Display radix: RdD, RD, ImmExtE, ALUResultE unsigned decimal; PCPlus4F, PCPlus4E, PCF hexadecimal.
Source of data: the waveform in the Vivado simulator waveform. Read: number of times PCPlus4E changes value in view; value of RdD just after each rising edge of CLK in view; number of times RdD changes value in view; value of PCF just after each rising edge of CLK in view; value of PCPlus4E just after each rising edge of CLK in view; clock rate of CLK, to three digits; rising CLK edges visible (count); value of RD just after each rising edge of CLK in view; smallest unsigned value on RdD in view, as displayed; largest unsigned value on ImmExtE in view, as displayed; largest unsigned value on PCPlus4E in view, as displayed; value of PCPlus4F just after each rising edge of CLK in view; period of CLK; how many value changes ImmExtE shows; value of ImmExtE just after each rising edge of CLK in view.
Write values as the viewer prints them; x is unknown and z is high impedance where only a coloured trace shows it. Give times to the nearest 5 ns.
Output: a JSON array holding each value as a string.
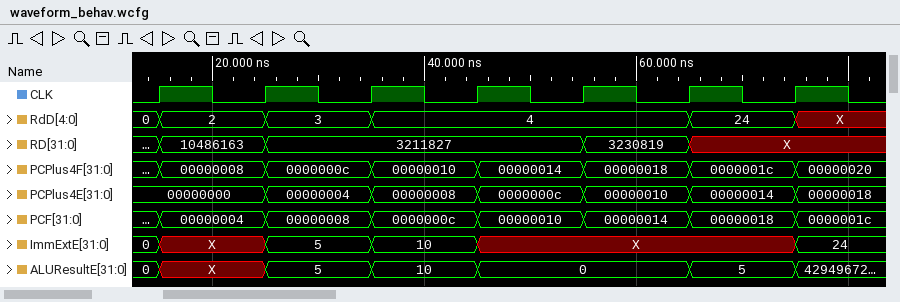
["6", "2, 3, 4, 4, 4, 24, X", "5", "00000004, 00000008, 0000000c, 00000010, 00000014, 00000018, 0000001c", "00000000, 00000004, 00000008, 0000000c, 00000010, 00000014, 00000018", "100 MHz", "7", "10486163, 3211827, 3211827, 3211827, 3230819, X, X", "0", "24", "00000018", "00000008, 0000000c, 00000010, 00000014, 00000018, 0000001c, 00000020", "10 ns", "5", "X, 5, 10, X, X, X, 24"]
